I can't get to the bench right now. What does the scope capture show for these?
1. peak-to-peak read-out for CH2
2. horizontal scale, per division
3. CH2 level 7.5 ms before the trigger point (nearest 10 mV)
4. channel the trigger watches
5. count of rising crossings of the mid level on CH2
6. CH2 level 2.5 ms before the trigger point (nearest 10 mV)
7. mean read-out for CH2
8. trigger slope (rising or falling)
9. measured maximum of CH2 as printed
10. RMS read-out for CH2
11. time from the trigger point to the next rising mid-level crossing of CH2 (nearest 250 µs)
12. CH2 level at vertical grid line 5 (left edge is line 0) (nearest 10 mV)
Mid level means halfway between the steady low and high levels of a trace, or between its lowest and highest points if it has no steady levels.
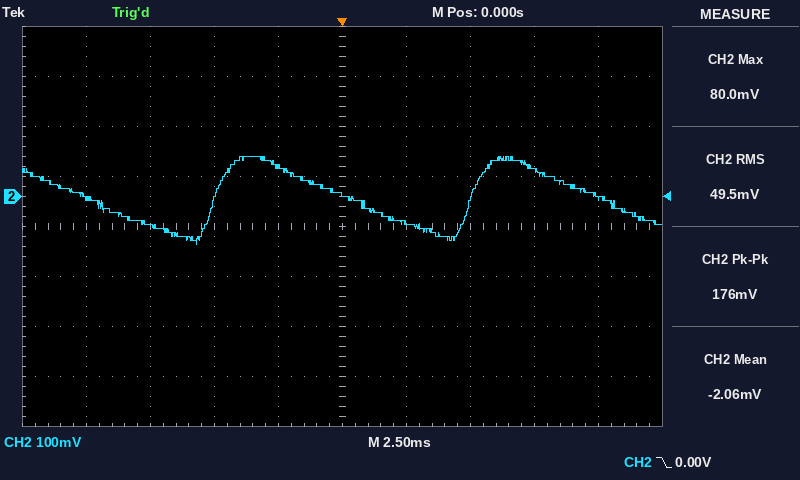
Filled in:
176 mV
2.5 ms
-60 mV
CH2
2
60 mV
-2.06 mV
falling
80.0 mV
49.5 mV
5.00 ms
0 mV
